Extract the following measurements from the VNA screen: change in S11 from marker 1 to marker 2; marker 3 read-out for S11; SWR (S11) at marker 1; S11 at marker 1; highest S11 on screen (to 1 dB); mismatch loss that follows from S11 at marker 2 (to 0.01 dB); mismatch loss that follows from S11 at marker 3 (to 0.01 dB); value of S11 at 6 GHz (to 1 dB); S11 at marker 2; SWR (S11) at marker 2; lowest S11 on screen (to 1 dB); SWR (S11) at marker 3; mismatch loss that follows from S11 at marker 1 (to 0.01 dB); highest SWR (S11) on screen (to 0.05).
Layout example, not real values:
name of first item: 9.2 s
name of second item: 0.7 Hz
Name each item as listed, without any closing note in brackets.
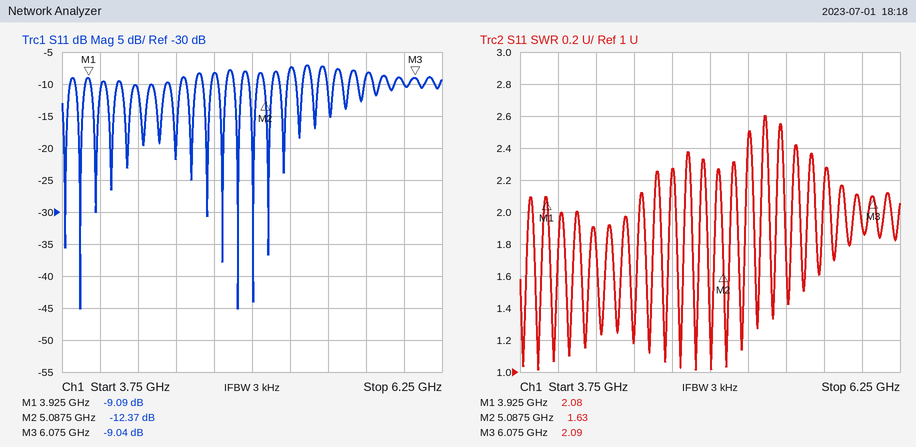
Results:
change in S11 from marker 1 to marker 2: -3.28 dB
marker 3 read-out for S11: -9.04 dB
SWR (S11) at marker 1: 2.08
S11 at marker 1: -9.09 dB
highest S11 on screen: -7 dB
mismatch loss that follows from S11 at marker 2: 0.26 dB
mismatch loss that follows from S11 at marker 3: 0.58 dB
value of S11 at 6 GHz: -10 dB
S11 at marker 2: -12.37 dB
SWR (S11) at marker 2: 1.63
lowest S11 on screen: -45 dB
SWR (S11) at marker 3: 2.09
mismatch loss that follows from S11 at marker 1: 0.57 dB
highest SWR (S11) on screen: 2.60
